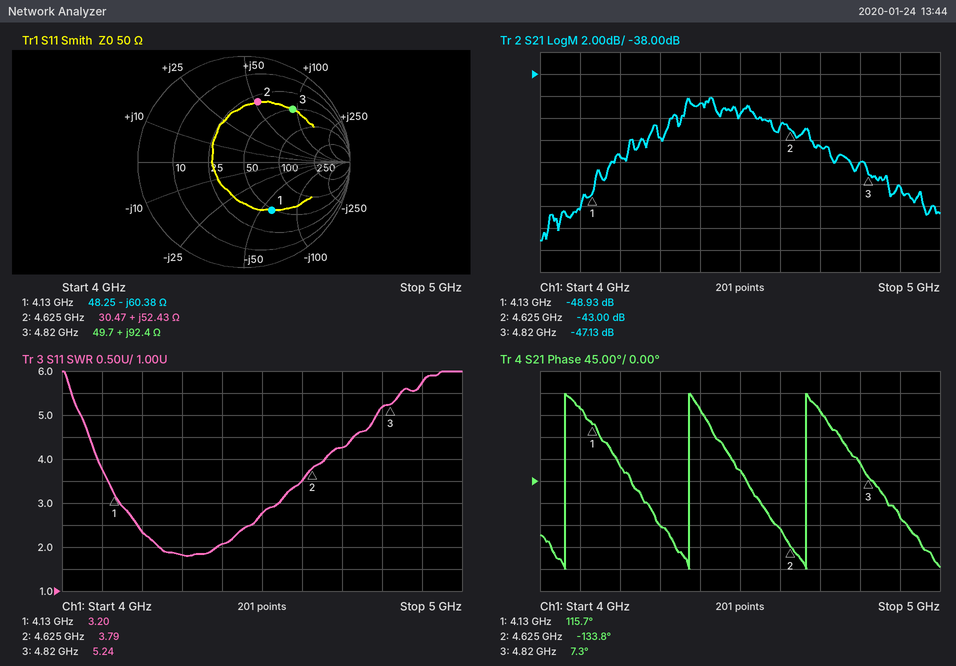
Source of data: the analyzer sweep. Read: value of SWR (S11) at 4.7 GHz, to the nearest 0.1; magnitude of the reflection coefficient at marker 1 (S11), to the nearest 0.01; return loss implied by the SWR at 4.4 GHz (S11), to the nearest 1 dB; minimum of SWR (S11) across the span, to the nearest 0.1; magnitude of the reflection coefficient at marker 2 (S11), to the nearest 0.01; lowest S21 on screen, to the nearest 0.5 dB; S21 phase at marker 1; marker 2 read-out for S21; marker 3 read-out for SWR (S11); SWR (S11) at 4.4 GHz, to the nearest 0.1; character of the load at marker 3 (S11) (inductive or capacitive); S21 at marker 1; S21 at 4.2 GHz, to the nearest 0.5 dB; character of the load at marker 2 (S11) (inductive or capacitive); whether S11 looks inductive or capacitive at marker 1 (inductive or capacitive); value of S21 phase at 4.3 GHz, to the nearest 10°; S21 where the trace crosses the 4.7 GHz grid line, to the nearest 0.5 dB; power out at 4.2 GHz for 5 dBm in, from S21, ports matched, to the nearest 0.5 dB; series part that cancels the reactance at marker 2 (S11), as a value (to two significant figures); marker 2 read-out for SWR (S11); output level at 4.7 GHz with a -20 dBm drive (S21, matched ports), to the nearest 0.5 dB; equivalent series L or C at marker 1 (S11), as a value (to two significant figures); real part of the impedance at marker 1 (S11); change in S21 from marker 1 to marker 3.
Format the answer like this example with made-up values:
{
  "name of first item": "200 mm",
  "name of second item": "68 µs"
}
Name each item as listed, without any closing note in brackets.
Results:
{
  "value of SWR (S11) at 4.7 GHz, to the nearest 0.1": "4.3",
  "magnitude of the reflection coefficient at marker 1 (S11), to the nearest 0.01": "0.52",
  "return loss implied by the SWR at 4.4 GHz (S11), to the nearest 1 dB": "9 dB",
  "minimum of SWR (S11) across the span, to the nearest 0.1": "1.8",
  "magnitude of the reflection coefficient at marker 2 (S11), to the nearest 0.01": "0.58",
  "lowest S21 on screen, to the nearest 0.5 dB": "-53.0 dB",
  "S21 phase at marker 1": "115.7°",
  "marker 2 read-out for S21": "-43.00 dB",
  "marker 3 read-out for SWR": "5.24",
  "SWR (S11) at 4.4 GHz, to the nearest 0.1": "2.1",
  "character of the load at marker 3 (S11)": "inductive",
  "S21 at marker 1": "-48.93 dB",
  "S21 at 4.2 GHz, to the nearest 0.5 dB": "-45.5 dB",
  "character of the load at marker 2 (S11)": "inductive",
  "whether S11 looks inductive or capacitive at marker 1": "capacitive",
  "value of S21 phase at 4.3 GHz, to the nearest 10°": "-90°",
  "S21 where the trace crosses the 4.7 GHz grid line, to the nearest 0.5 dB": "-44.5 dB",
  "power out at 4.2 GHz for 5 dBm in, from S21, ports matched, to the nearest 0.5 dB": "-40.5 dBm",
  "series part that cancels the reactance at marker 2 (S11), as a value": "660 fF",
  "marker 2 read-out for SWR": "3.79",
  "output level at 4.7 GHz with a -20 dBm drive (S21, matched ports), to the nearest 0.5 dB": "-64.5 dBm",
  "equivalent series L or C at marker 1 (S11), as a value": "640 fF",
  "real part of the impedance at marker 1": "48.25 Ω",
  "change in S21 from marker 1 to marker 3": "1.80 dB"
}
